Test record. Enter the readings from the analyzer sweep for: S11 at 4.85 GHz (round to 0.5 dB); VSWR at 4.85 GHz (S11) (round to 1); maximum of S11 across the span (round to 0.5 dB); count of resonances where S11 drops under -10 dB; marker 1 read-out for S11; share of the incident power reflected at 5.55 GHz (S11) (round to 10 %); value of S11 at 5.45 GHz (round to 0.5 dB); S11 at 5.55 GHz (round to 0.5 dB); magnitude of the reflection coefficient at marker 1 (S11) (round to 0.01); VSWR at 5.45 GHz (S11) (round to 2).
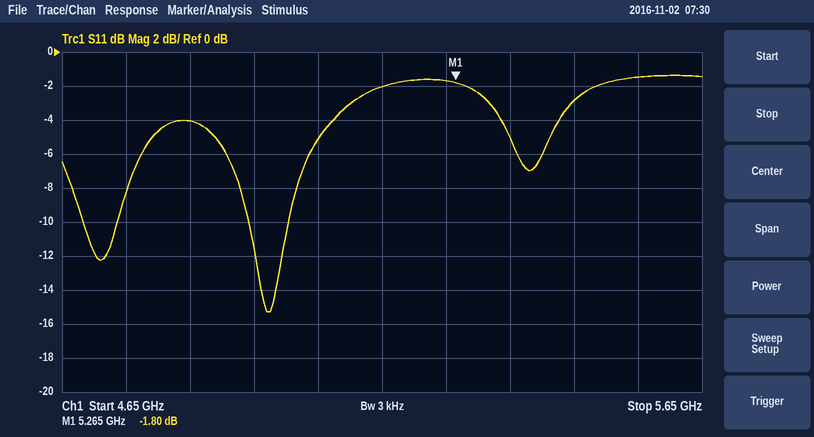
-4.0 dB
4
-1.5 dB
2
-1.80 dB
70 %
-3.0 dB
-1.5 dB
0.81
6
